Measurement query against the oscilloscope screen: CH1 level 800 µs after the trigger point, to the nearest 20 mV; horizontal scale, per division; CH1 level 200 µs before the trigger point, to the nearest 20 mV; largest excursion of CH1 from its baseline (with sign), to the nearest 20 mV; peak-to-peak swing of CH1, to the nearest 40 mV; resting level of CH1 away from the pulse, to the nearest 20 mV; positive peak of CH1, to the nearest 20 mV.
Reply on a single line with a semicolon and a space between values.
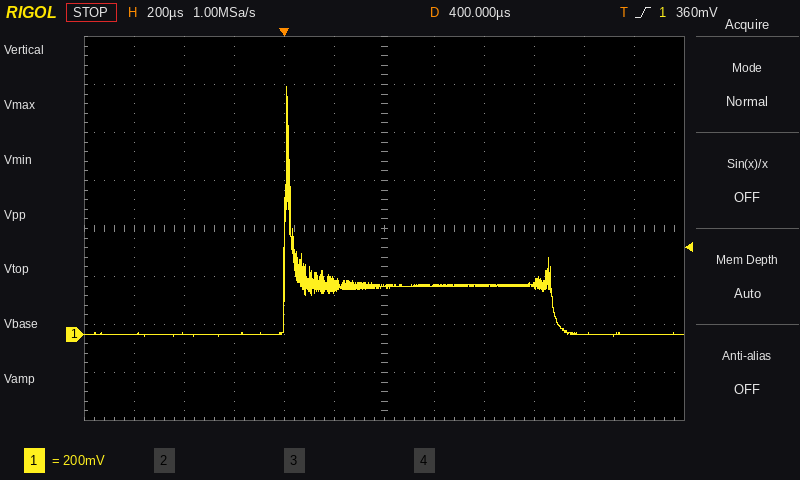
200 mV; 200 µs; 0 mV; +1.04 V; 1.04 V; 0 mV; 1.04 V
